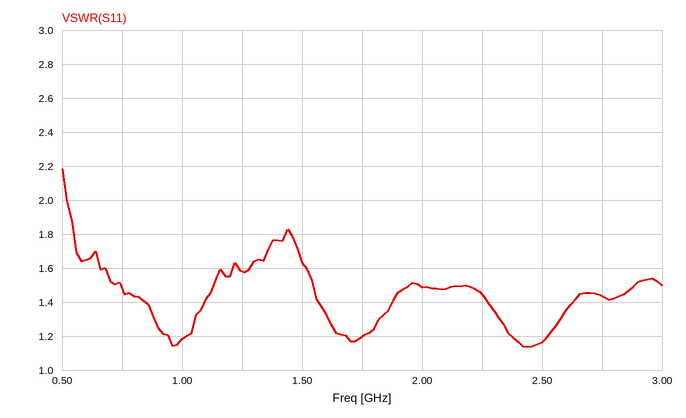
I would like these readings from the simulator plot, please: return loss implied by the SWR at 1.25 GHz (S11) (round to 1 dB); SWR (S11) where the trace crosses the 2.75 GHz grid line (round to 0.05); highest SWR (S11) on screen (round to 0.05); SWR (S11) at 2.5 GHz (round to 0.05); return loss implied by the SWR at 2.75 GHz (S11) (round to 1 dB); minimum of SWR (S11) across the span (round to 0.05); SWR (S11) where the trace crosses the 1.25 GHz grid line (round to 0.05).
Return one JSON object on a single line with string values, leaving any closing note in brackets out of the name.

{"return loss implied by the SWR at 1.25 GHz (S11)": "13 dB", "SWR (S11) where the trace crosses the 2.75 GHz grid line": "1.45", "highest SWR (S11) on screen": "2.20", "SWR (S11) at 2.5 GHz": "1.15", "return loss implied by the SWR at 2.75 GHz (S11)": "15 dB", "minimum of SWR (S11) across the span": "1.15", "SWR (S11) where the trace crosses the 1.25 GHz grid line": "1.60"}
